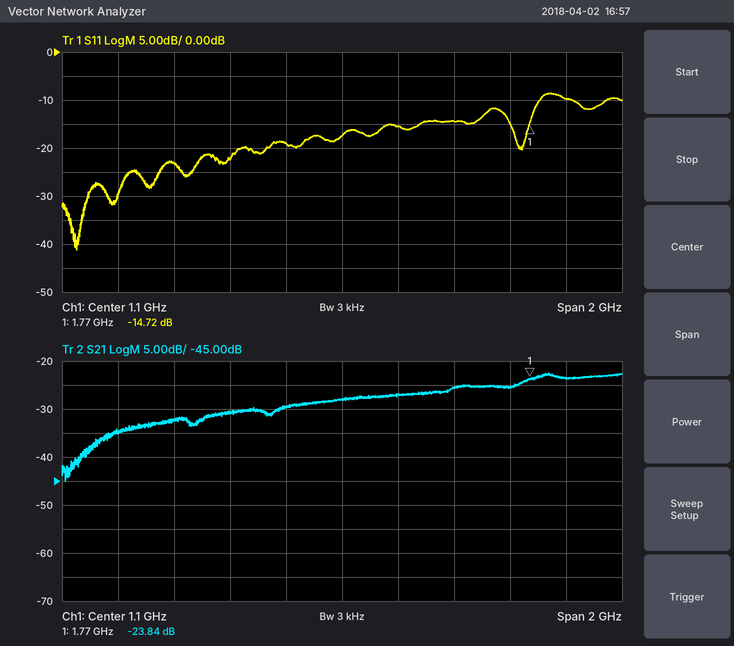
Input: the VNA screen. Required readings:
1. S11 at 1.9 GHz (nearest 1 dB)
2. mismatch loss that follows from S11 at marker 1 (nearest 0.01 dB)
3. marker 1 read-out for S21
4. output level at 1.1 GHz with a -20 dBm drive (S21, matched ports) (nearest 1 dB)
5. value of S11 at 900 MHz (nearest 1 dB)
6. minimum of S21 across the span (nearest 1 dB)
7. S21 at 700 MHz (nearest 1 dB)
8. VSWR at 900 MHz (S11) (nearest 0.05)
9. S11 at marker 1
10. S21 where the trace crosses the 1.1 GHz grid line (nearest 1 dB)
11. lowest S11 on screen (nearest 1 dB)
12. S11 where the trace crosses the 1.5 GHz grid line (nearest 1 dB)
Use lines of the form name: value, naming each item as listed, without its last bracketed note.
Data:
S11 at 1.9 GHz: -10 dB
mismatch loss that follows from S11 at marker 1: 0.15 dB
marker 1 read-out for S21: -23.84 dB
output level at 1.1 GHz with a -20 dBm drive (S21, matched ports): -48 dBm
value of S11 at 900 MHz: -19 dB
minimum of S21 across the span: -45 dB
S21 at 700 MHz: -31 dB
VSWR at 900 MHz (S11): 1.25
S11 at marker 1: -14.72 dB
S21 where the trace crosses the 1.1 GHz grid line: -28 dB
lowest S11 on screen: -41 dB
S11 where the trace crosses the 1.5 GHz grid line: -14 dB
